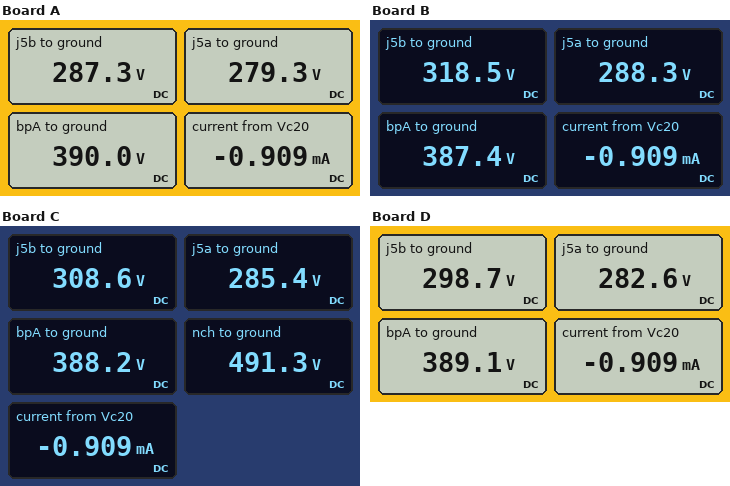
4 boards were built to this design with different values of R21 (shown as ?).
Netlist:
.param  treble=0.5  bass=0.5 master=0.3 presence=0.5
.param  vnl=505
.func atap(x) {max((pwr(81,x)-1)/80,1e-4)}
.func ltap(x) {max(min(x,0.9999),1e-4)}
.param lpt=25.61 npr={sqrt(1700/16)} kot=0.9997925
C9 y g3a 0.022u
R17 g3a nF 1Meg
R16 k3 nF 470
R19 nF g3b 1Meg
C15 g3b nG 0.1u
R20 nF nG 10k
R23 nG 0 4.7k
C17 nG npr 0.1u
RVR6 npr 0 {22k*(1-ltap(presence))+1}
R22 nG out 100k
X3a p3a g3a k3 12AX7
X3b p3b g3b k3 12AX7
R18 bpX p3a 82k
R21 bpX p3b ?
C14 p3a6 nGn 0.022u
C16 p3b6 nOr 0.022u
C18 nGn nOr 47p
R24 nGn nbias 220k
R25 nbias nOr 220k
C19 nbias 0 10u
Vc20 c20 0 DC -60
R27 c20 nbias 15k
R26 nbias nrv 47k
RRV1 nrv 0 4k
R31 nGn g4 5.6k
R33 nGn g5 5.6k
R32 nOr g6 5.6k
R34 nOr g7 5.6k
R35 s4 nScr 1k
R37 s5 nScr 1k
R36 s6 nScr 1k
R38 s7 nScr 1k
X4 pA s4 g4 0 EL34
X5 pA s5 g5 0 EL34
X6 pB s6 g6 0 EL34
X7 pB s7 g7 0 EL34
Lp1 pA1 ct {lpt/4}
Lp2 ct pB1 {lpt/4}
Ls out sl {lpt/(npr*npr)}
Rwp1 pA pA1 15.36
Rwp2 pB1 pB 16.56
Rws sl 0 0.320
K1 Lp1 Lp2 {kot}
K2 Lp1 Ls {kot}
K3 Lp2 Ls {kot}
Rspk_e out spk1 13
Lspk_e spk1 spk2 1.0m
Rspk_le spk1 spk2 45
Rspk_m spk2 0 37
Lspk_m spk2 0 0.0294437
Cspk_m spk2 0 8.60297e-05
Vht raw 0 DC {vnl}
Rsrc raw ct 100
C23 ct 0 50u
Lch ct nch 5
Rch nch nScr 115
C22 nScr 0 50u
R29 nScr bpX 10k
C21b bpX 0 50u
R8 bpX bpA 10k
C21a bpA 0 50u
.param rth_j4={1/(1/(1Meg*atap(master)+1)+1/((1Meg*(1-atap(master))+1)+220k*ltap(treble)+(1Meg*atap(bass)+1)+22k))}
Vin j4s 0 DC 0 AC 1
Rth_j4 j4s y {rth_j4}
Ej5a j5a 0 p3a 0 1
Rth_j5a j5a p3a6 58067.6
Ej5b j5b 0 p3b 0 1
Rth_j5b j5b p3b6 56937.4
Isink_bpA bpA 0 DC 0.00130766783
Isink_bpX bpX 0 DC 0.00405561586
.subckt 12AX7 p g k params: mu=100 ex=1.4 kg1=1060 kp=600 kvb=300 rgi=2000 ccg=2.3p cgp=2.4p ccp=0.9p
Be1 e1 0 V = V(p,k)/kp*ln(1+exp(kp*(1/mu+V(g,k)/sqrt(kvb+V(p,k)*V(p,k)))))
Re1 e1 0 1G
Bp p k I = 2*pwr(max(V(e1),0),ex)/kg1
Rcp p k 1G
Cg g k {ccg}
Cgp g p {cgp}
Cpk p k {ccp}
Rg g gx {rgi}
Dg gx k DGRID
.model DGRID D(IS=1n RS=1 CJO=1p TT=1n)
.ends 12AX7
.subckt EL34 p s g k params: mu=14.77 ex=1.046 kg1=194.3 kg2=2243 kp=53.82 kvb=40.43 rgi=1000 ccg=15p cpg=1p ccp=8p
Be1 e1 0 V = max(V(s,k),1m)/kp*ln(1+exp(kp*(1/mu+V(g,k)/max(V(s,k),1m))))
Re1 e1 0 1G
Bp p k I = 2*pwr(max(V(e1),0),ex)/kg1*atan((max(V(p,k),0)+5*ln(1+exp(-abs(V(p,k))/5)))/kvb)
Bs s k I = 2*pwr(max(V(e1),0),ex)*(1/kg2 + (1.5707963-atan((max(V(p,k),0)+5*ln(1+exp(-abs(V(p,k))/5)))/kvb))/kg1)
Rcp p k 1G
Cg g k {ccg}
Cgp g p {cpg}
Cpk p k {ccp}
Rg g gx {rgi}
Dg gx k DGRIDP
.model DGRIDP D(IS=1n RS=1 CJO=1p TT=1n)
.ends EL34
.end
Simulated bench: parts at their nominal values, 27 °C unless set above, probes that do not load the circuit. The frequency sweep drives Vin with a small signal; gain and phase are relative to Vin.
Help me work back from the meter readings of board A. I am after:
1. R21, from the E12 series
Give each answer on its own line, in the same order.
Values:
68 kΩ
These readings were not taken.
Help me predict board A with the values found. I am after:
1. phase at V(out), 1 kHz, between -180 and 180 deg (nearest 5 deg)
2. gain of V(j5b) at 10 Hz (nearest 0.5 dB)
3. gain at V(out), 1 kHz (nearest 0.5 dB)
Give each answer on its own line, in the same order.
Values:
10 deg
27.0 dB
21.0 dB
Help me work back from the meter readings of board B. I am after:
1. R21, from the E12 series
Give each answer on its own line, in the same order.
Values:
39 kΩ
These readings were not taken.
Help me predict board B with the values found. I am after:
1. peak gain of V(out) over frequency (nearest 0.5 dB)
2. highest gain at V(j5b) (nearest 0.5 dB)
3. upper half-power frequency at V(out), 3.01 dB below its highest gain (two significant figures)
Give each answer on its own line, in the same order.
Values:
26.5 dB
23.5 dB
70 kHz
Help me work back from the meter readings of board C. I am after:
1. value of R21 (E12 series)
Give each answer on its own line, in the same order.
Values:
47 kΩ
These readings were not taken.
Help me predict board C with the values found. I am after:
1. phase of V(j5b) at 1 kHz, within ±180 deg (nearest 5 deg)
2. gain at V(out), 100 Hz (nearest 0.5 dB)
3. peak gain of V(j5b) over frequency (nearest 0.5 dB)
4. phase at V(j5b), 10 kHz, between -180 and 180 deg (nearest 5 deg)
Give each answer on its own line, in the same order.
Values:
-5 deg
25.0 dB
25.0 dB
-5 deg
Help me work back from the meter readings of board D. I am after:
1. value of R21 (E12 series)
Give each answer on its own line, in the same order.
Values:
56 kΩ
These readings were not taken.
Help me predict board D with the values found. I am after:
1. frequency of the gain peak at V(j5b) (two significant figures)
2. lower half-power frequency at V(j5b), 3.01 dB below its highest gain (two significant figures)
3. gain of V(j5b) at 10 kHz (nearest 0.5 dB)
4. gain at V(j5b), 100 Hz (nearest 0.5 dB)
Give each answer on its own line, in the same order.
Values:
13 Hz
4.4 Hz
17.0 dB
16.0 dB
